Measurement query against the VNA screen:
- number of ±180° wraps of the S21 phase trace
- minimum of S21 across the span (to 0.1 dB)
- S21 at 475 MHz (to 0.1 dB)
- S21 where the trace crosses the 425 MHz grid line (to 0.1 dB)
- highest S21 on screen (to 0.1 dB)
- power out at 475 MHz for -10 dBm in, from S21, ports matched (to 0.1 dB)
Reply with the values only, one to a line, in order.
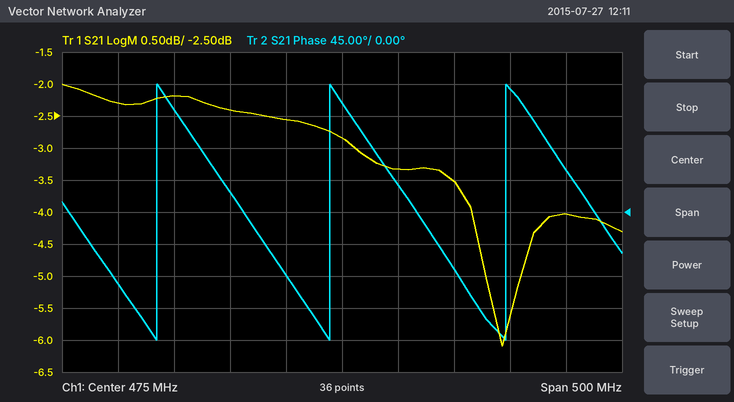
3
-6.1 dB
-2.8 dB
-2.6 dB
-2.0 dB
-12.8 dBm
